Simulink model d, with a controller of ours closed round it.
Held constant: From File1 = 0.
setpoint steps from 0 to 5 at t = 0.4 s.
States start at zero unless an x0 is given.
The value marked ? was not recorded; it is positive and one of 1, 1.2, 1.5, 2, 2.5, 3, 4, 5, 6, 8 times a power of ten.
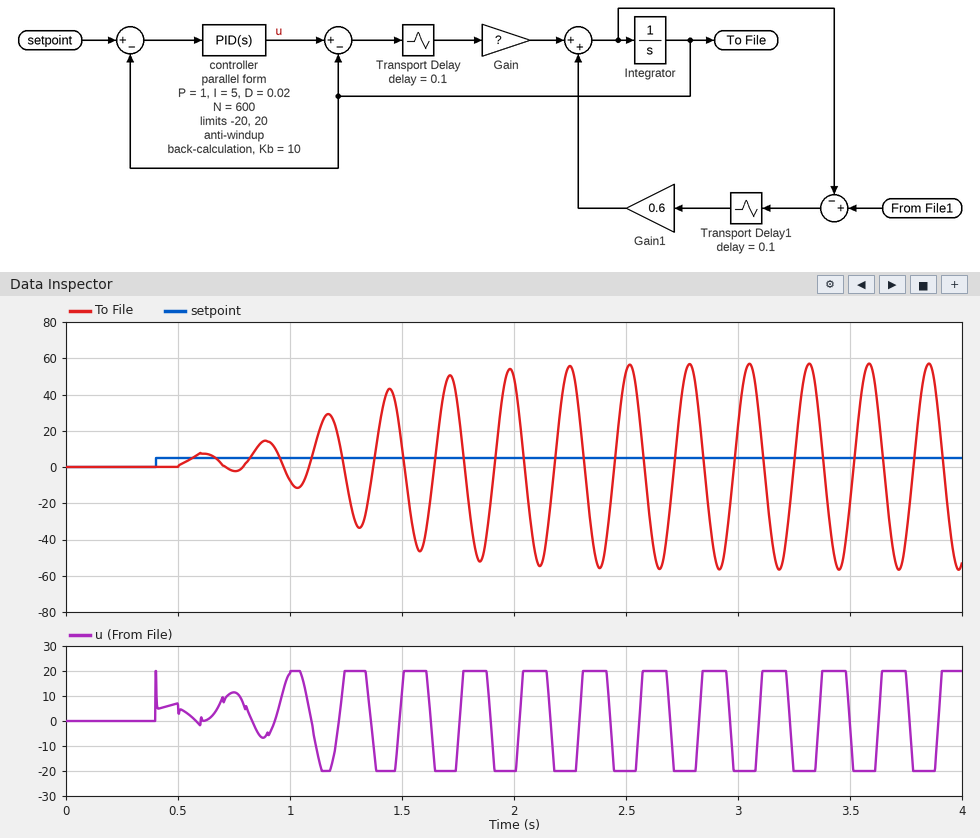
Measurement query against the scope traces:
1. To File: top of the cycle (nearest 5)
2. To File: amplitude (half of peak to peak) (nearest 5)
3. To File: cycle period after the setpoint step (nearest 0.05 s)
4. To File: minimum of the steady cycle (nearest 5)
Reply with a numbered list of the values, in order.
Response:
1. 55
2. 55
3. 0.25 s
4. -55
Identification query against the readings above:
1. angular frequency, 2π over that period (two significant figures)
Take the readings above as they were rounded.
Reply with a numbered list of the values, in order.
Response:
1. 25 rad/s
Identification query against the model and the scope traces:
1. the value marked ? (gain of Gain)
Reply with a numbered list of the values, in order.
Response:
1. 12
